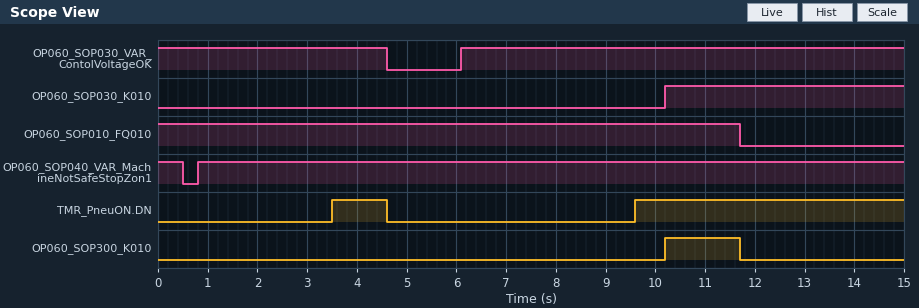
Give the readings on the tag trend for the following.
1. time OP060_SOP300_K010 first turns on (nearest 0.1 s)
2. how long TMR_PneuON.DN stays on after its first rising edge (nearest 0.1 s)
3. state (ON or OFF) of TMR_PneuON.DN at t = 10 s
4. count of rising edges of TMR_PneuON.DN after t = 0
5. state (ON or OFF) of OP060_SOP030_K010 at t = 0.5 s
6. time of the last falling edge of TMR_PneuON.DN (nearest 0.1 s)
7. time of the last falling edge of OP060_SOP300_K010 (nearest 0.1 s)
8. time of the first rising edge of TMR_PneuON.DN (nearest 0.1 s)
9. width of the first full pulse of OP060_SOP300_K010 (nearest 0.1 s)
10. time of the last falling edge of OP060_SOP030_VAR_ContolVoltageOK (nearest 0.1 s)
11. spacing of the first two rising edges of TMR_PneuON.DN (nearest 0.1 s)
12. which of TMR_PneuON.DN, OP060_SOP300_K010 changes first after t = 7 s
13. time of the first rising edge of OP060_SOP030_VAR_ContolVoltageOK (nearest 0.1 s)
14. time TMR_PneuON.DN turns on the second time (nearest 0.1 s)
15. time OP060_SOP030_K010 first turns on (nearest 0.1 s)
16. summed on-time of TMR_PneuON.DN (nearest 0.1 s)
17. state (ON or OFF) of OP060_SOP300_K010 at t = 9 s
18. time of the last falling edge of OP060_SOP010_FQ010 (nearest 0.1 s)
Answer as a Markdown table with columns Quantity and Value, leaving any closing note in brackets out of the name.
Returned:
| Quantity | Value |
|---|---|
| time OP060_SOP300_K010 first turns on | 10.2 s |
| how long TMR_PneuON.DN stays on after its first rising edge | 1.1 s |
| state (ON or OFF) of TMR_PneuON.DN at t = 10 s | ON |
| count of rising edges of TMR_PneuON.DN after t = 0 | 2 |
| state (ON or OFF) of OP060_SOP030_K010 at t = 0.5 s | OFF |
| time of the last falling edge of TMR_PneuON.DN | 4.6 s |
| time of the last falling edge of OP060_SOP300_K010 | 11.7 s |
| time of the first rising edge of TMR_PneuON.DN | 3.5 s |
| width of the first full pulse of OP060_SOP300_K010 | 1.5 s |
| time of the last falling edge of OP060_SOP030_VAR_ContolVoltageOK | 4.6 s |
| spacing of the first two rising edges of TMR_PneuON.DN | 6.1 s |
| which of TMR_PneuON.DN, OP060_SOP300_K010 changes first after t = 7 s | TMR_PneuON.DN |
| time of the first rising edge of OP060_SOP030_VAR_ContolVoltageOK | 6.1 s |
| time TMR_PneuON.DN turns on the second time | 9.6 s |
| time OP060_SOP030_K010 first turns on | 10.2 s |
| summed on-time of TMR_PneuON.DN | 6.5 s |
| state (ON or OFF) of OP060_SOP300_K010 at t = 9 s | OFF |
| time of the last falling edge of OP060_SOP010_FQ010 | 11.7 s |
